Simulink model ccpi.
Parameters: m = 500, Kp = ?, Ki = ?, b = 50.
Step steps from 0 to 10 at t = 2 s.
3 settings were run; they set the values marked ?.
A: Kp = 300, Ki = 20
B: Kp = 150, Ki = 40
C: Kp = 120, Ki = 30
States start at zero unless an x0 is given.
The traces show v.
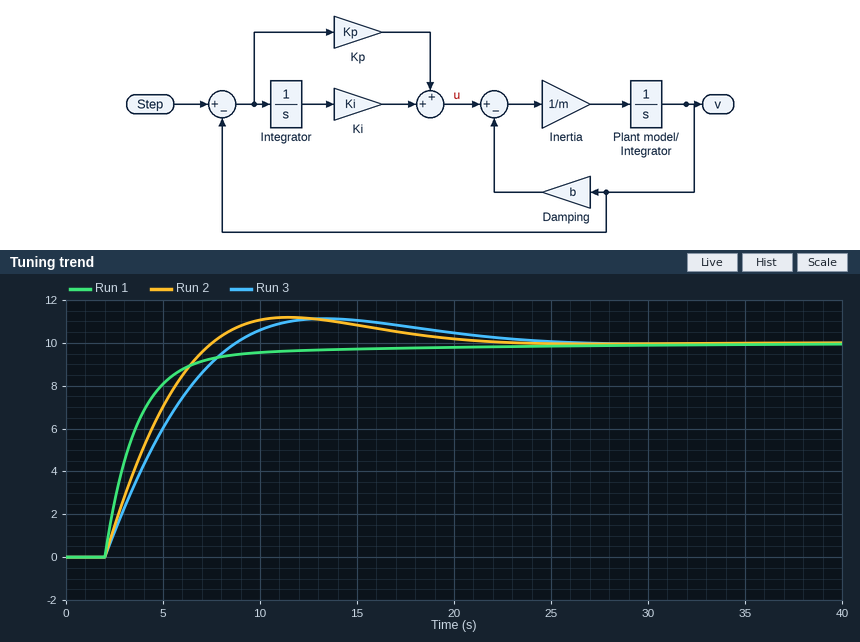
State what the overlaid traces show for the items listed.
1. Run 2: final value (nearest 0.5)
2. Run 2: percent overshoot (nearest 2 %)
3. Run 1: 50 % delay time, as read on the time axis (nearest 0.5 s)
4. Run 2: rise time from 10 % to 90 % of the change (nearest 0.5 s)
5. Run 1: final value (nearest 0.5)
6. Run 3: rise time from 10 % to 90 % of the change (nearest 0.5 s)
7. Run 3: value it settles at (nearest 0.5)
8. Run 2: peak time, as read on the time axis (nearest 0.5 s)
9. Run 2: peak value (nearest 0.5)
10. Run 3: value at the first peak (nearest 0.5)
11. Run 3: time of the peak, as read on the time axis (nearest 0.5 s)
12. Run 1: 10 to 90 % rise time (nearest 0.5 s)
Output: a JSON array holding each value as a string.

["10.0", "12 %", "3.0 s", "4.0 s", "10.0", "5.0 s", "10.0", "11.5 s", "11.0", "11.0", "13.5 s", "4.5 s"]
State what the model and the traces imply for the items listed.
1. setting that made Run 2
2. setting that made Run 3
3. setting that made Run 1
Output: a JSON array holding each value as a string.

["B", "C", "A"]
